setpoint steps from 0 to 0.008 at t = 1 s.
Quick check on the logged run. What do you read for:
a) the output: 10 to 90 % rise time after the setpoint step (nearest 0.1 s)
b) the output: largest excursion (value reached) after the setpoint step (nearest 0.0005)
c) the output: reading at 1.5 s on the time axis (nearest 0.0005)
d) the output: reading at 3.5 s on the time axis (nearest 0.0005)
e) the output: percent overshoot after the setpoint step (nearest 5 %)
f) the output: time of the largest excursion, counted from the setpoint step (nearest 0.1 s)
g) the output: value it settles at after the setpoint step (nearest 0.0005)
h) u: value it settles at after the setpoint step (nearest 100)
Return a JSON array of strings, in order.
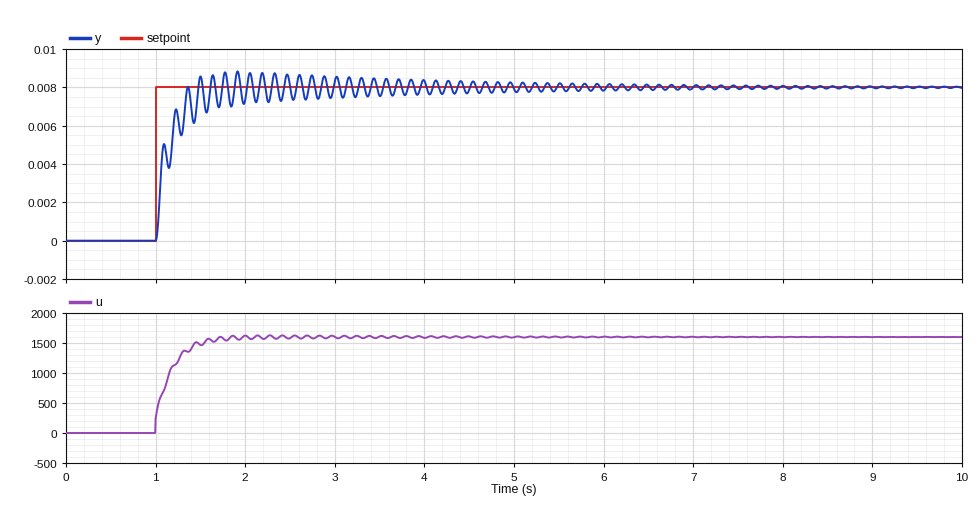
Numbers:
["0.3 s", "0.0090", "0.0085", "0.0075", "10 %", "0.9 s", "0.0080", "1600"]
